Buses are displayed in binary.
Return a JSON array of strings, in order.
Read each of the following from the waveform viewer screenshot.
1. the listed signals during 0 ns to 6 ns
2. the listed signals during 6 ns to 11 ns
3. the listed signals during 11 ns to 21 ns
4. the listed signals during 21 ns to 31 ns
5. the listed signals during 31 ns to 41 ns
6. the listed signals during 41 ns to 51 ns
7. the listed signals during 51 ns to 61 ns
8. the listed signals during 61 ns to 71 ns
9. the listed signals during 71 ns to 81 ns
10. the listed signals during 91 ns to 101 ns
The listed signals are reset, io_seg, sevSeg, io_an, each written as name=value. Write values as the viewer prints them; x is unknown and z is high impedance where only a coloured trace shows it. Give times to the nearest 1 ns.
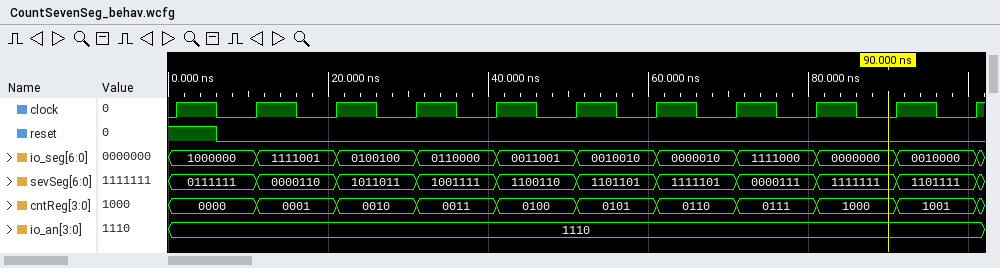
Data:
["reset=1, io_seg=1000000, sevSeg=0111111, io_an=1110", "reset=0, io_seg=1000000, sevSeg=0111111, io_an=1110", "reset=0, io_seg=1111001, sevSeg=0000110, io_an=1110", "reset=0, io_seg=0100100, sevSeg=1011011, io_an=1110", "reset=0, io_seg=0110000, sevSeg=1001111, io_an=1110", "reset=0, io_seg=0011001, sevSeg=1100110, io_an=1110", "reset=0, io_seg=0010010, sevSeg=1101101, io_an=1110", "reset=0, io_seg=0000010, sevSeg=1111101, io_an=1110", "reset=0, io_seg=1111000, sevSeg=0000111, io_an=1110", "reset=0, io_seg=0010000, sevSeg=1101111, io_an=1110"]
